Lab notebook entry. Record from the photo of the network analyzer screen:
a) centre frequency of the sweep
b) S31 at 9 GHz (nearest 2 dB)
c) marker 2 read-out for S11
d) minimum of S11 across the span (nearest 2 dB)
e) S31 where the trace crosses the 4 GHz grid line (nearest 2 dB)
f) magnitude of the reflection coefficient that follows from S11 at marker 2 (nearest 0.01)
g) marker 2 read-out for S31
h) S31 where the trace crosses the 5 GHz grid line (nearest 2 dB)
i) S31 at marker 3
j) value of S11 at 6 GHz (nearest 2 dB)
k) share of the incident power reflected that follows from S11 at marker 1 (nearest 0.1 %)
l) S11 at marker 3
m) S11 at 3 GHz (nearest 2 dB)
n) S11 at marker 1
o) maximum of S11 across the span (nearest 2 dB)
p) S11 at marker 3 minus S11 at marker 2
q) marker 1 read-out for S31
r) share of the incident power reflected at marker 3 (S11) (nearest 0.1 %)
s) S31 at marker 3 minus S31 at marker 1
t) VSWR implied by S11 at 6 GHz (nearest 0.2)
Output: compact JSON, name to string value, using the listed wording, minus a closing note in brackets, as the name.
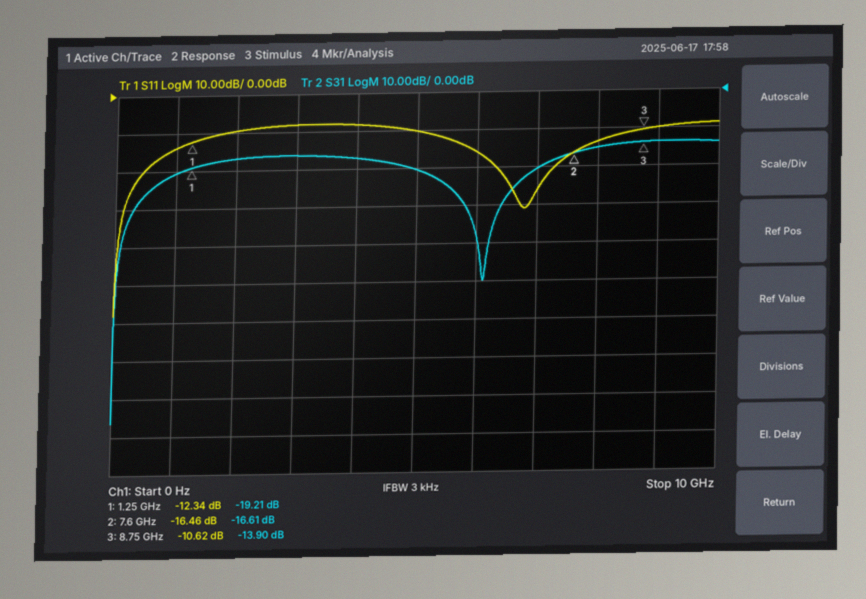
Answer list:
{"centre frequency of the sweep": "5 GHz", "S31 at 9 GHz": "-14 dB", "marker 2 read-out for S11": "-16.46 dB", "minimum of S11 across the span": "-58 dB", "S31 where the trace crosses the 4 GHz grid line": "-18 dB", "magnitude of the reflection coefficient that follows from S11 at marker 2": "0.15", "marker 2 read-out for S31": "-16.61 dB", "S31 where the trace crosses the 5 GHz grid line": "-20 dB", "S31 at marker 3": "-13.90 dB", "value of S11 at 6 GHz": "-16 dB", "share of the incident power reflected that follows from S11 at marker 1": "5.8 %", "S11 at marker 3": "-10.62 dB", "S11 at 3 GHz": "-8 dB", "S11 at marker 1": "-12.34 dB", "maximum of S11 across the span": "-8 dB", "S11 at marker 3 minus S11 at marker 2": "5.84 dB", "marker 1 read-out for S31": "-19.21 dB", "share of the incident power reflected at marker 3 (S11)": "8.7 %", "S31 at marker 3 minus S31 at marker 1": "5.31 dB", "VSWR implied by S11 at 6 GHz": "1.4"}
